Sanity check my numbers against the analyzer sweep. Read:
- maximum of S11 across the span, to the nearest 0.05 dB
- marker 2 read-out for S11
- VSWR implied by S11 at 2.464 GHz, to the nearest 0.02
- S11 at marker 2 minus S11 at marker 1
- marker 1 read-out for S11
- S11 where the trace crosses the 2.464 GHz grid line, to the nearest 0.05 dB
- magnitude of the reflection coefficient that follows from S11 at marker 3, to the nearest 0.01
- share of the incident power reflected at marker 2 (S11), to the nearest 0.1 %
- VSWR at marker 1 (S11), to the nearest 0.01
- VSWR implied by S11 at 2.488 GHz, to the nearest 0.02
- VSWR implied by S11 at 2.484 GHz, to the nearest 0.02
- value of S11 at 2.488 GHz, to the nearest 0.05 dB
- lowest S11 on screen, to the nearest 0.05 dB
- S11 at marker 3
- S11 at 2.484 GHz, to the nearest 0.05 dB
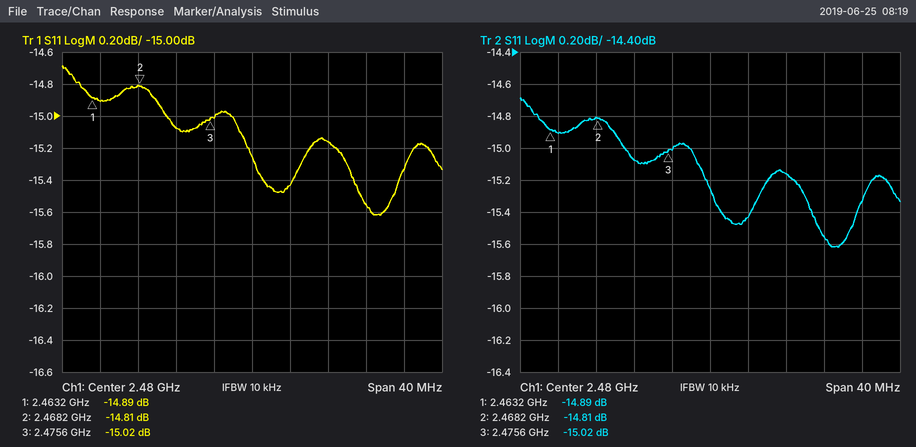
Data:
-14.70 dB
-14.81 dB
1.44
0.08 dB
-14.89 dB
-14.90 dB
0.18
3.3 %
1.44
1.42
1.40
-15.15 dB
-15.60 dB
-15.02 dB
-15.45 dB
